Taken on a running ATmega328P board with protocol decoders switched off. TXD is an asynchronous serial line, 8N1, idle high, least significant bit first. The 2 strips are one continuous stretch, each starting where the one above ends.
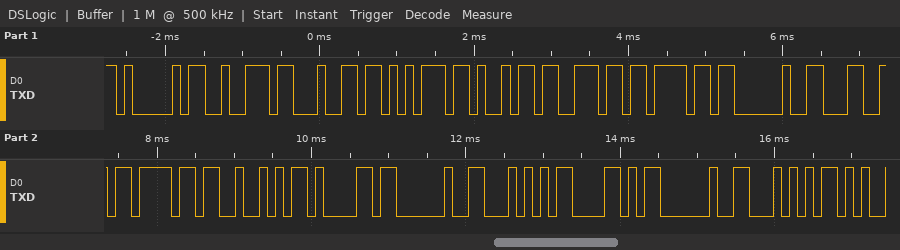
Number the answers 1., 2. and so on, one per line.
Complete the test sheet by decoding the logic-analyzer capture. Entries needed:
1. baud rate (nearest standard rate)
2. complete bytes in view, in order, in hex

1. 9600 baud
2. 41 72 64 75 69 6E 6F 20 4C 6F 52 61 20 54 58 20 54
